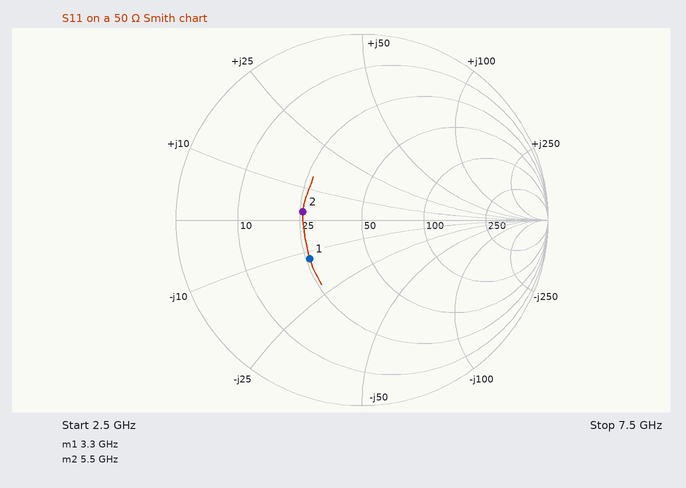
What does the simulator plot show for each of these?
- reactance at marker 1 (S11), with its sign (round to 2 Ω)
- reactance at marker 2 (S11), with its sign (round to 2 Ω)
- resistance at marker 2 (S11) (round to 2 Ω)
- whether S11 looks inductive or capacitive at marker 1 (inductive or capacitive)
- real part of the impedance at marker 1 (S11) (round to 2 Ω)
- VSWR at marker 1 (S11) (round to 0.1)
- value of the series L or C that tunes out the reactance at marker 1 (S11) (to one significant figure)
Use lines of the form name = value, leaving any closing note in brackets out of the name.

reactance at marker 1 (S11), with its sign = -12 Ω
reactance at marker 2 (S11), with its sign = +2 Ω
resistance at marker 2 (S11) = 26 Ω
whether S11 looks inductive or capacitive at marker 1 = capacitive
real part of the impedance at marker 1 (S11) = 26 Ω
VSWR at marker 1 (S11) = 2.1
value of the series L or C that tunes out the reactance at marker 1 (S11) = 600 pH
